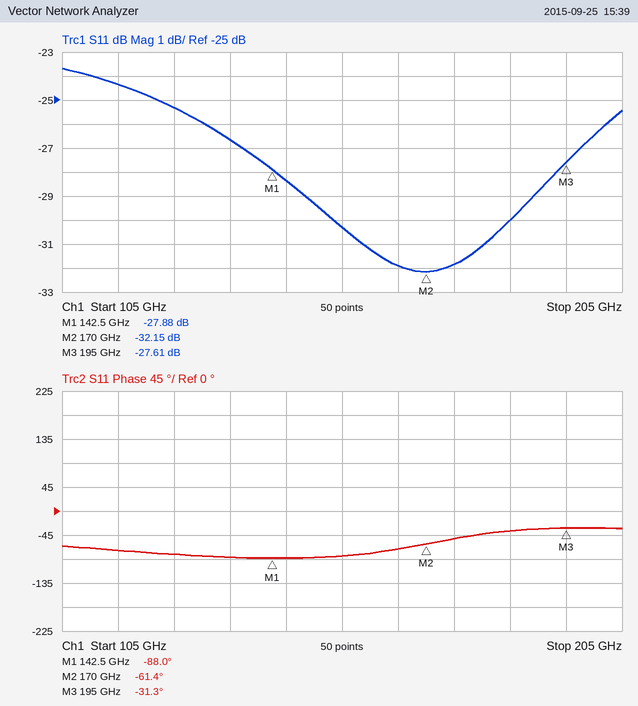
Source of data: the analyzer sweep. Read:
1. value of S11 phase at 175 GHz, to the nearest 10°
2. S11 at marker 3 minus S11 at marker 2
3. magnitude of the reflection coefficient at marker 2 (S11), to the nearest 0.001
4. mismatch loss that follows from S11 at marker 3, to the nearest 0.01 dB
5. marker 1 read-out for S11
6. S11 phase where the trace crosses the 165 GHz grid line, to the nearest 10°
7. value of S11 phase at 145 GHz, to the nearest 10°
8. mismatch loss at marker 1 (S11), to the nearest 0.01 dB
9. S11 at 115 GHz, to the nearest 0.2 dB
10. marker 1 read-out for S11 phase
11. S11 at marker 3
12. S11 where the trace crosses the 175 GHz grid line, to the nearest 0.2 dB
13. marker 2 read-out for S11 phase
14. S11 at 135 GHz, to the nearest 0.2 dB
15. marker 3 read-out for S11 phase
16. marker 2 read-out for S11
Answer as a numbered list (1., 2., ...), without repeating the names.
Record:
1. -50°
2. 4.54 dB
3. 0.025
4. 0.01 dB
5. -27.88 dB
6. -70°
7. -90°
8. 0.01 dB
9. -24.4 dB
10. -88.0°
11. -27.61 dB
12. -31.8 dB
13. -61.4°
14. -26.6 dB
15. -31.3°
16. -32.15 dB
